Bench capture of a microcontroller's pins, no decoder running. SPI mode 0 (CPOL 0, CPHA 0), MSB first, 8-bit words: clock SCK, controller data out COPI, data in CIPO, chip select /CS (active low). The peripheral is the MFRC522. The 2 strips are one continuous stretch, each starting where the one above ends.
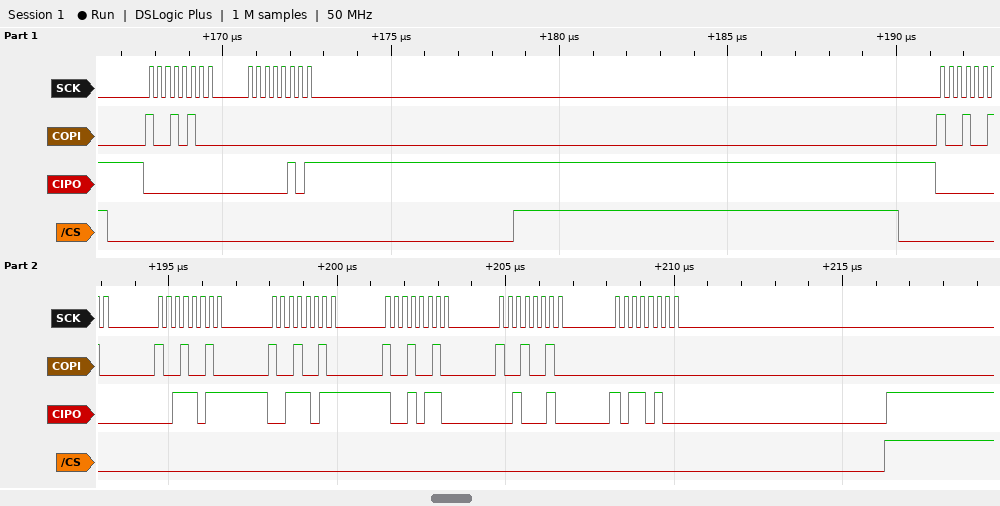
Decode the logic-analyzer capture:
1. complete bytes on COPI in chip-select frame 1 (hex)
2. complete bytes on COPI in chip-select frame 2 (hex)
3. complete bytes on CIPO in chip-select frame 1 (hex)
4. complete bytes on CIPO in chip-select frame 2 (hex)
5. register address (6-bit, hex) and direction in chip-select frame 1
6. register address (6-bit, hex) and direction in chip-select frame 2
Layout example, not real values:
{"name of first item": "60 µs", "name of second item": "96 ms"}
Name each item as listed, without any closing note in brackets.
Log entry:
{"complete bytes on COPI in chip-select frame 1": "94 00", "complete bytes on COPI in chip-select frame 2": "92 92 92 92 92 00", "complete bytes on CIPO in chip-select frame 1": "00 05", "complete bytes on CIPO in chip-select frame 2": "00 3B 3B 96 22 B4", "register address (6-bit, hex) and direction in chip-select frame 1": "0x0A read", "register address (6-bit, hex) and direction in chip-select frame 2": "0x09 read"}
